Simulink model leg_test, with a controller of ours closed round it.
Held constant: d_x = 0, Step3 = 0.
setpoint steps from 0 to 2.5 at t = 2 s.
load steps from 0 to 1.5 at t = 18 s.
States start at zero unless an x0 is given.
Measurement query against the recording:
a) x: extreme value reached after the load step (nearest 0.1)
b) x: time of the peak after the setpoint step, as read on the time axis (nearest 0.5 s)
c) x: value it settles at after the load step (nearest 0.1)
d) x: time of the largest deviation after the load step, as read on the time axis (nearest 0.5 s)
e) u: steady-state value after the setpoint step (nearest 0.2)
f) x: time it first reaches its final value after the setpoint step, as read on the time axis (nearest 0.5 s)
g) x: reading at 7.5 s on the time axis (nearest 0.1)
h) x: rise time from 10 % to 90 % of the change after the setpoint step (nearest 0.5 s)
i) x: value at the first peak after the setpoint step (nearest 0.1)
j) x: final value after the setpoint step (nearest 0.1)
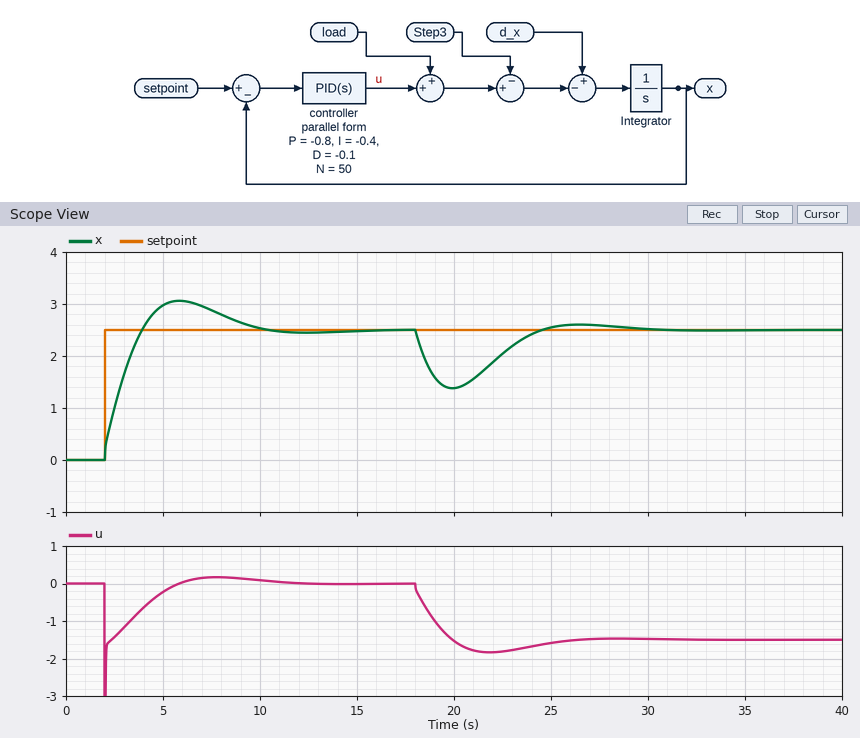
1.4
6.0 s
2.5
20.0 s
0.0
4.0 s
2.9
1.5 s
3.1
2.5
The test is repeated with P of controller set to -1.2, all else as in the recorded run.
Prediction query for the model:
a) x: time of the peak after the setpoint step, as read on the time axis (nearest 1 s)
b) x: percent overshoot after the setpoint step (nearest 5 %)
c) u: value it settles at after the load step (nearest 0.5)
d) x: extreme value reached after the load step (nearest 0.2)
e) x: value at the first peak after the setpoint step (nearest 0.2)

5 s
15 %
-1.5
1.6
2.8
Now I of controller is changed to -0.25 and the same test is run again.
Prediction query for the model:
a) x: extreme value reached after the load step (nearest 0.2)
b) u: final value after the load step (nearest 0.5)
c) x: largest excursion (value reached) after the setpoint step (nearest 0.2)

1.2
-1.5
3.0
